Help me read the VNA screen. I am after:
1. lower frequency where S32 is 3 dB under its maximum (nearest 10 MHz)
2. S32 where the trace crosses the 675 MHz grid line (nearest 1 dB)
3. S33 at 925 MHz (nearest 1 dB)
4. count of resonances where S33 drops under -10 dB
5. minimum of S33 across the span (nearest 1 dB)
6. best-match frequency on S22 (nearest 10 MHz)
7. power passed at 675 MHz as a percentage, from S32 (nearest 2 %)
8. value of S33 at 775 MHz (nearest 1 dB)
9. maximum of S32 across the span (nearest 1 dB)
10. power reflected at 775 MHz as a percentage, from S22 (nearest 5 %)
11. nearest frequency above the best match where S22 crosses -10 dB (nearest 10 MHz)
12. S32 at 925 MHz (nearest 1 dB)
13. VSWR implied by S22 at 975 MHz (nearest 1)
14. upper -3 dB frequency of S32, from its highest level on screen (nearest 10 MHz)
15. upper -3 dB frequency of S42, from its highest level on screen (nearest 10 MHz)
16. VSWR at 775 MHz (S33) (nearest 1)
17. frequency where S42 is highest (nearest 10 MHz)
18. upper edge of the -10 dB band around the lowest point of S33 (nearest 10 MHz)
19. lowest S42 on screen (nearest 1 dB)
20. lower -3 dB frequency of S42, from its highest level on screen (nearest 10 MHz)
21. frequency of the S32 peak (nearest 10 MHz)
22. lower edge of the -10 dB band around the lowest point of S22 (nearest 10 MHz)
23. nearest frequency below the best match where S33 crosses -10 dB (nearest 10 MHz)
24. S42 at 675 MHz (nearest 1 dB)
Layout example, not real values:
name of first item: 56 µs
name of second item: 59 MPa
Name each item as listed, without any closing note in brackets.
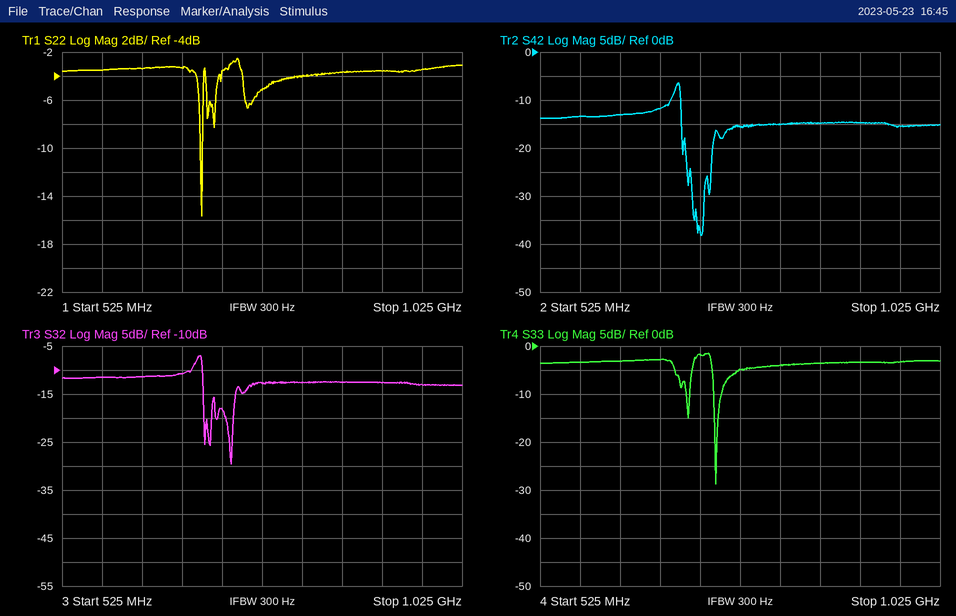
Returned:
lower frequency where S32 is 3 dB under its maximum: 690 MHz
S32 where the trace crosses the 675 MHz grid line: -11 dB
S33 at 925 MHz: -3 dB
count of resonances where S33 drops under -10 dB: 2
minimum of S33 across the span: -29 dB
best-match frequency on S22: 700 MHz
power passed at 675 MHz as a percentage, from S32: 8 %
value of S33 at 775 MHz: -5 dB
maximum of S32 across the span: -7 dB
power reflected at 775 MHz as a percentage, from S22: 30 %
nearest frequency above the best match where S22 crosses -10 dB: 700 MHz
S32 at 925 MHz: -13 dB
VSWR implied by S22 at 975 MHz: 5
upper -3 dB frequency of S32, from its highest level on screen: 700 MHz
upper -3 dB frequency of S42, from its highest level on screen: 700 MHz
VSWR at 775 MHz (S33): 4
frequency where S42 is highest: 700 MHz
upper edge of the -10 dB band around the lowest point of S33: 750 MHz
lowest S42 on screen: -38 dB
lower -3 dB frequency of S42, from its highest level on screen: 690 MHz
frequency of the S32 peak: 700 MHz
lower edge of the -10 dB band around the lowest point of S22: 700 MHz
nearest frequency below the best match where S33 crosses -10 dB: 740 MHz
S42 at 675 MHz: -12 dB
